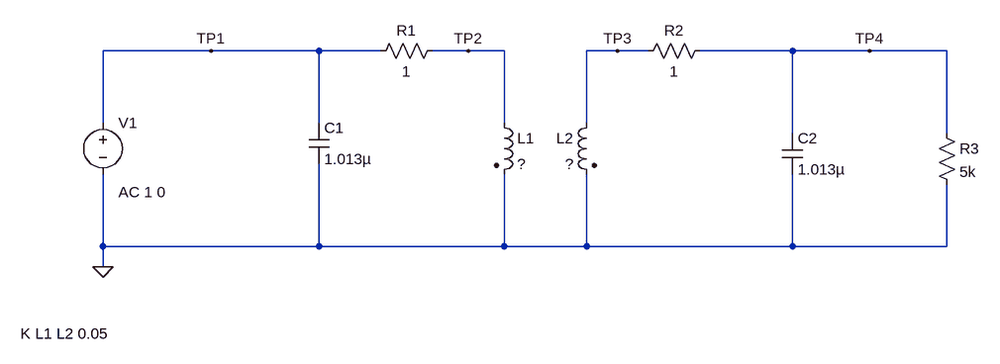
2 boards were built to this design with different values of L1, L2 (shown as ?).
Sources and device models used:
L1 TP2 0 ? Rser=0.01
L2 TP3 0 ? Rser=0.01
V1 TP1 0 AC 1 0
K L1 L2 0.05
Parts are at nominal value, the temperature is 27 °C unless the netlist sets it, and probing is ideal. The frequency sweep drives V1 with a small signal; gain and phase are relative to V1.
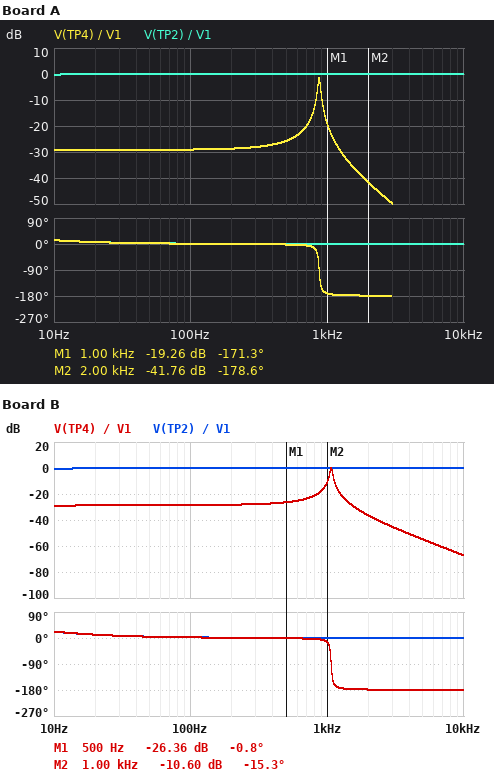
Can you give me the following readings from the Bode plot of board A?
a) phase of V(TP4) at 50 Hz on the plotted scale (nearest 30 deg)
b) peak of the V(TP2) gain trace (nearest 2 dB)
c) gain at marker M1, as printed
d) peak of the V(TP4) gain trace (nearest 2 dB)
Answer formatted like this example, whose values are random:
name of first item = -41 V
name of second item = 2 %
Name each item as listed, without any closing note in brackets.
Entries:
phase of V(TP4) at 50 Hz on the plotted scale = 0 deg
peak of the V(TP2) gain trace = 0 dB
gain at marker M1, as printed = -19.26 dB
peak of the V(TP4) gain trace = -2 dB
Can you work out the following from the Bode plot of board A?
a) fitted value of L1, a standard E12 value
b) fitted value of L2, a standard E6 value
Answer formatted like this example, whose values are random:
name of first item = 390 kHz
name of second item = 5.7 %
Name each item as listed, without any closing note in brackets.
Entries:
fitted value of L1, a standard E12 value = 68 mH
fitted value of L2, a standard E6 value = 33 mH
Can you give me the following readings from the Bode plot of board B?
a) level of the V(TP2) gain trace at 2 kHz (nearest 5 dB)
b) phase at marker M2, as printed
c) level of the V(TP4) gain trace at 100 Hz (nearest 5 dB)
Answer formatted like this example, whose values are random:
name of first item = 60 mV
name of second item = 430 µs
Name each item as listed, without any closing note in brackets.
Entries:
level of the V(TP2) gain trace at 2 kHz = 0 dB
phase at marker M2, as printed = -15.3 deg
level of the V(TP4) gain trace at 100 Hz = -30 dB
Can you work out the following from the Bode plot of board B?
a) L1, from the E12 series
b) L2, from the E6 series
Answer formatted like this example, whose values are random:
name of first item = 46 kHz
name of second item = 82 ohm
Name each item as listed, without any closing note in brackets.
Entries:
L1, from the E12 series = 39 mH
L2, from the E6 series = 22 mH
